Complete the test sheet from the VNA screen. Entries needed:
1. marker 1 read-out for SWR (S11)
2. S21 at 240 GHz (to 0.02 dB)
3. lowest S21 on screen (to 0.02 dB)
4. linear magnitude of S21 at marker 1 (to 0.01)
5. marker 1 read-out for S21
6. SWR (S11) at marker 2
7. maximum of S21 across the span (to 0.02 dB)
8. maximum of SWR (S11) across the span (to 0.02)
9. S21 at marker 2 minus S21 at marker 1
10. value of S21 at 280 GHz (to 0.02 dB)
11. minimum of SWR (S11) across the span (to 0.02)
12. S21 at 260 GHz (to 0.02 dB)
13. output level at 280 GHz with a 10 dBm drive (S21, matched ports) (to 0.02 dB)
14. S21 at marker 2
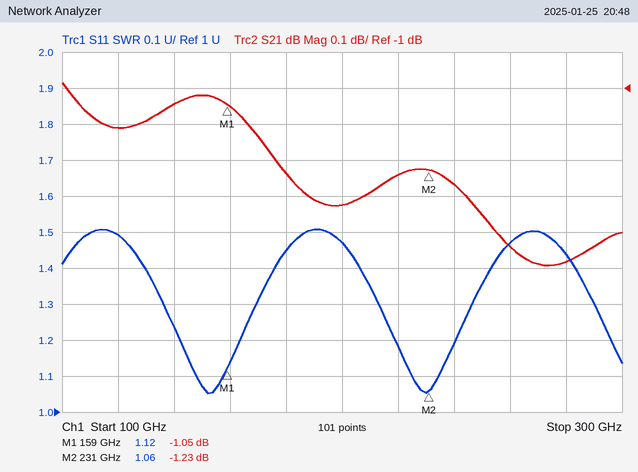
1.12
-1.26 dB
-1.50 dB
0.89
-1.05 dB
1.06
-0.98 dB
1.50
-0.18 dB
-1.48 dB
1.06
-1.44 dB
8.52 dBm
-1.23 dB
